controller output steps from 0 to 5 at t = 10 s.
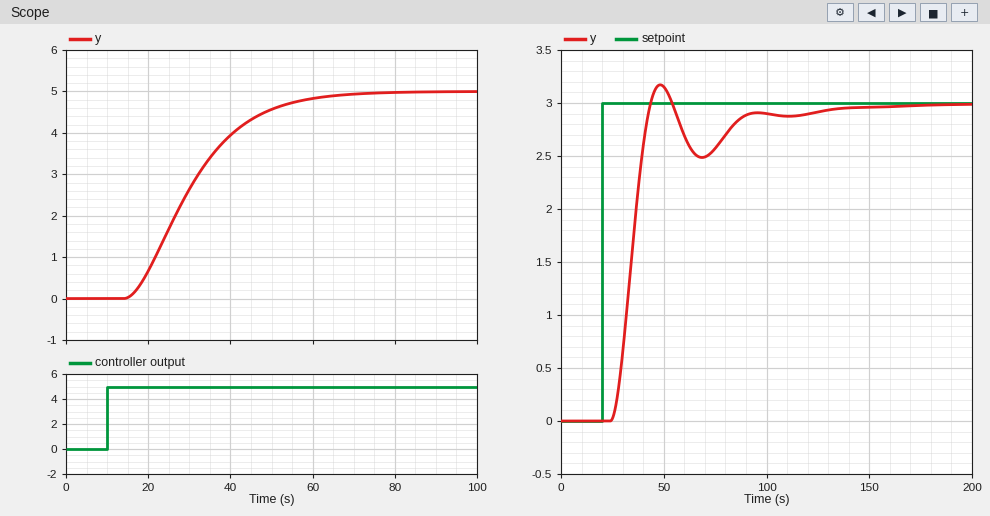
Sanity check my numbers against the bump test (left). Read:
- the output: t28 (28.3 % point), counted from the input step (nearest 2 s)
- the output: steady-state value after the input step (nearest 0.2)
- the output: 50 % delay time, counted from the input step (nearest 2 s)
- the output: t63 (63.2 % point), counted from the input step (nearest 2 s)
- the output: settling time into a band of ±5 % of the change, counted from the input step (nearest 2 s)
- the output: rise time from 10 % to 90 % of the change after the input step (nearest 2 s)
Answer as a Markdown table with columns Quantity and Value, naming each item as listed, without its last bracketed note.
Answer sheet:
| Quantity | Value |
|---|---|
| the output: t28 (28.3 % point), counted from the input step | 14 s |
| the output: steady-state value after the input step | 5.0 |
| the output: 50 % delay time, counted from the input step | 20 s |
| the output: t63 (63.2 % point), counted from the input step | 24 s |
| the output: settling time into a band of ±5 % of the change, counted from the input step | 46 s |
| the output: rise time from 10 % to 90 % of the change after the input step | 30 s |
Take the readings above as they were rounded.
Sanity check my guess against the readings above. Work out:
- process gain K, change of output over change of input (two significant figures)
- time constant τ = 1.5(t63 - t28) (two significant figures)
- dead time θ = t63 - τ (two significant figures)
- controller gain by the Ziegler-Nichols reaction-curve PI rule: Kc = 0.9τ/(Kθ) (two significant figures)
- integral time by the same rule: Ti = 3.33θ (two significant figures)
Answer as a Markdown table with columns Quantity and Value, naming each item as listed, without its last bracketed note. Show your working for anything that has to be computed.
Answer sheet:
| Quantity | Value |
|---|---|
| process gain K, change of output over change of input | (5 - 0) / 5 = 1.0 |
| time constant τ = 1.5(t63 - t28) | 1.5 × (24 - 14) = 15 s |
| dead time θ = t63 - τ | 24 - 15 = 9.0 s |
| controller gain by the Ziegler-Nichols reaction-curve PI rule: Kc = 0.9τ/(Kθ) | 0.9 × 15 / (1 × 9) = 1.5 |
| integral time by the same rule: Ti = 3.33θ | 3.33 × 9 = 30 s |
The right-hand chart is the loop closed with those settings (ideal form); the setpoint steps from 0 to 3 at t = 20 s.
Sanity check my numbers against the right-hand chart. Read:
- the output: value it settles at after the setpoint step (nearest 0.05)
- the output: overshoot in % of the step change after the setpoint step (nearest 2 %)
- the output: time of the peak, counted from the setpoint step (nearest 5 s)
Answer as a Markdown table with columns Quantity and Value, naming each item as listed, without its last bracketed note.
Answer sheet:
| Quantity | Value |
|---|---|
| the output: value it settles at after the setpoint step | 3.00 |
| the output: overshoot in % of the step change after the setpoint step | 6 % |
| the output: time of the peak, counted from the setpoint step | 30 s |
